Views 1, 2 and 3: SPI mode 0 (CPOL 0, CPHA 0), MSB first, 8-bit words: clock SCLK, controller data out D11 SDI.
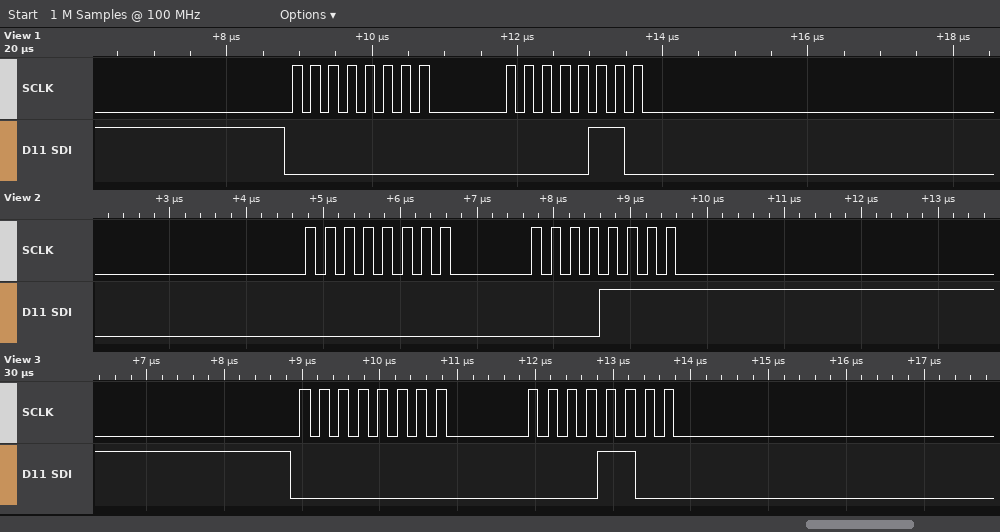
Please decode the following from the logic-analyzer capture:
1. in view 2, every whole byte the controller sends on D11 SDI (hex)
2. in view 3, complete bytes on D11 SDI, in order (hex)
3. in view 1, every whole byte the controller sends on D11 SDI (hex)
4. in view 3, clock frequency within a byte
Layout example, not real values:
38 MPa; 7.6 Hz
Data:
00 0F; 00 0C; 00 06; 4 MHz
